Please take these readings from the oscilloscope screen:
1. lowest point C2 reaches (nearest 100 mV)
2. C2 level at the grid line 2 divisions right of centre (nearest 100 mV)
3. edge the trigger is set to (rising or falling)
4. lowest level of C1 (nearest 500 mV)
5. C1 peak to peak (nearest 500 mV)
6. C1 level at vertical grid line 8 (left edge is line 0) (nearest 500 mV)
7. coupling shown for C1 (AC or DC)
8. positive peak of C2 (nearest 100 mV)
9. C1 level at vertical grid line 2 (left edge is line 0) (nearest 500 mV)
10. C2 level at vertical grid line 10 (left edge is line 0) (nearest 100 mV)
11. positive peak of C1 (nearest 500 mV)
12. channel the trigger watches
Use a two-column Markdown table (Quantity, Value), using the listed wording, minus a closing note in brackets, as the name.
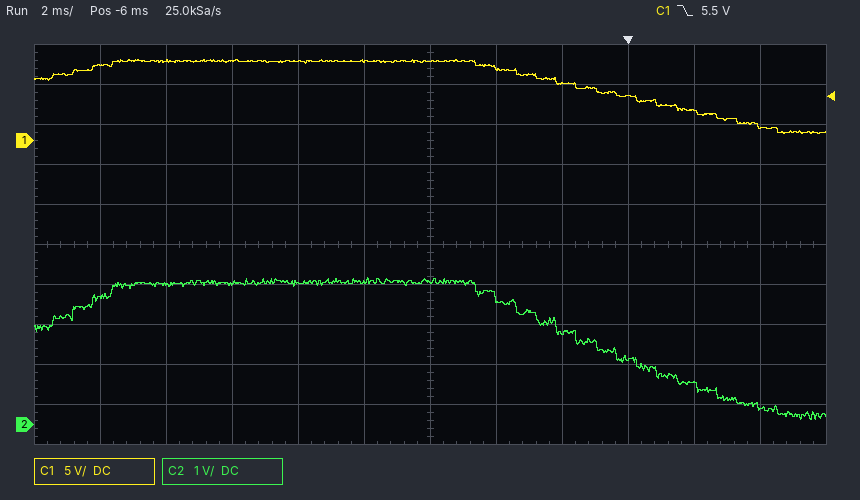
| Quantity | Value |
|---|---|
| lowest point C2 reaches | 100 mV |
| C2 level at the grid line 2 divisions right of centre | 2.3 V |
| edge the trigger is set to | falling |
| lowest level of C1 | 1.0 V |
| C1 peak to peak | 9.0 V |
| C1 level at vertical grid line 8 (left edge is line 0) | 7.0 V |
| coupling shown for C1 | DC |
| positive peak of C2 | 3.7 V |
| C1 level at vertical grid line 2 (left edge is line 0) | 10.0 V |
| C2 level at vertical grid line 10 (left edge is line 0) | 1.0 V |
| positive peak of C1 | 10.0 V |
| channel the trigger watches | C1 |
